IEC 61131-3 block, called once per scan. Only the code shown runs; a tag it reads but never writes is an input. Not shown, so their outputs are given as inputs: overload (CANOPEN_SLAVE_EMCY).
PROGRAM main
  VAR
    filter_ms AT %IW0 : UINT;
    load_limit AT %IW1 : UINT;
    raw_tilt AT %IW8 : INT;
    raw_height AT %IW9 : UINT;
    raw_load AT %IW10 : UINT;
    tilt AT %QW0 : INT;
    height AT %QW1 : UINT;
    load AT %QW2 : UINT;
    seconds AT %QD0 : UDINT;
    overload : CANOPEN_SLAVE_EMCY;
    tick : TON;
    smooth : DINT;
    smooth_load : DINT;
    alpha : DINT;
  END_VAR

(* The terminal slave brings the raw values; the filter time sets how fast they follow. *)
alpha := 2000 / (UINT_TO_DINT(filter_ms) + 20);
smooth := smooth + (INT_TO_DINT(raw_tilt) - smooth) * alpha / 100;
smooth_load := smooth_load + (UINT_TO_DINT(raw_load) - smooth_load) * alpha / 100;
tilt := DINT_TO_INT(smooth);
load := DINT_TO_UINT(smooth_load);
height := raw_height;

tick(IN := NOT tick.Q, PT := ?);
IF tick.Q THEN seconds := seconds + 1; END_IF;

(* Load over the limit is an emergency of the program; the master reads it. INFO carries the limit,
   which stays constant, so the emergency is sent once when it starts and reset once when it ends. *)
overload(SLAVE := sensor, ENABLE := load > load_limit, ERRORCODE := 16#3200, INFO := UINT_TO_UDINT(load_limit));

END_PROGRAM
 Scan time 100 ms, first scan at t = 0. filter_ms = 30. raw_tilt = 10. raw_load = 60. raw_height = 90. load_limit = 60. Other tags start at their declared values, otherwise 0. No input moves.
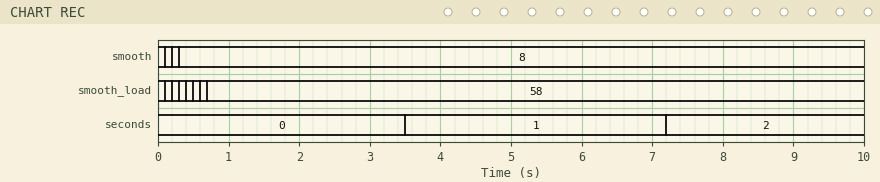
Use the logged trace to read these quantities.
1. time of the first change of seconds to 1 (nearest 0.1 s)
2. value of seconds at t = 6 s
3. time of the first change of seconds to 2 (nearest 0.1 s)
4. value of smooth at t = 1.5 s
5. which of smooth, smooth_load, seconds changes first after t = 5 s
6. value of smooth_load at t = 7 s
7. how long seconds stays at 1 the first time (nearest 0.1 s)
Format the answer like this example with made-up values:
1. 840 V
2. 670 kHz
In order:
1. 3.5 s
2. 1
3. 7.2 s
4. 8
5. seconds
6. 58
7. 3.7 s
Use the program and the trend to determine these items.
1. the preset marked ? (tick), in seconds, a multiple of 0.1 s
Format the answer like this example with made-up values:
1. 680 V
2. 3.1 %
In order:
1. 3.5 s
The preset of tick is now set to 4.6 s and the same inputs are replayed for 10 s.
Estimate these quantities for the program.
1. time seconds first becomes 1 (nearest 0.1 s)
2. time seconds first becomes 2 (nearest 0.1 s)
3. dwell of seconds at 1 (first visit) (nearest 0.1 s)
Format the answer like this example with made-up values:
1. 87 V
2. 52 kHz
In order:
1. 4.6 s
2. 9.4 s
3. 4.8 s
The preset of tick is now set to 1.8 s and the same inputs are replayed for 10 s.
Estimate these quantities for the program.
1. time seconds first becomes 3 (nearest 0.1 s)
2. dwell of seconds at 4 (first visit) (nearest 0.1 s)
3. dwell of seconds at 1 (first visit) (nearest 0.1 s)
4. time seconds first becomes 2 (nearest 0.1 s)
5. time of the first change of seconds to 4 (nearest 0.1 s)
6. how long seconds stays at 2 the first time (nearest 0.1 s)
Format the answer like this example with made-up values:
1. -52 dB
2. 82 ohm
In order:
1. 5.8 s
2. 2.0 s
3. 2.0 s
4. 3.8 s
5. 7.8 s
6. 2.0 s
